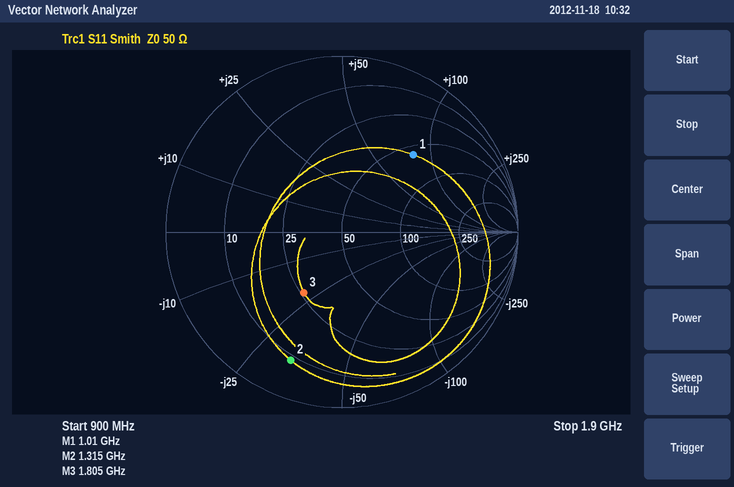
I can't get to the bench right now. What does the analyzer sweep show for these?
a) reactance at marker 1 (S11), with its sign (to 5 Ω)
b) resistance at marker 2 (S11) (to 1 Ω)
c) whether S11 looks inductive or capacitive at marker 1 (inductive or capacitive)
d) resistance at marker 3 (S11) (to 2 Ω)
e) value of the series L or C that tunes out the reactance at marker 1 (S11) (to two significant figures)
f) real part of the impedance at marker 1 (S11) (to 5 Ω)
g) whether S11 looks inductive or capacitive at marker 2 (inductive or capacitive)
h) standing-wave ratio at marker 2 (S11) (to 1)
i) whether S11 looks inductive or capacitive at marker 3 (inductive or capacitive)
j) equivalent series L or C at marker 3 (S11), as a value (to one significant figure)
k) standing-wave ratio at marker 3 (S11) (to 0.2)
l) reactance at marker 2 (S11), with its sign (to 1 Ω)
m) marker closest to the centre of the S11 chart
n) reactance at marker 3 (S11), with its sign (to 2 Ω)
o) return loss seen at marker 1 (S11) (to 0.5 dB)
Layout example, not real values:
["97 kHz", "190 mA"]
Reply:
["+80 Ω", "9 Ω", "inductive", "26 Ω", "2.0 pF", "60 Ω", "capacitive", "8", "capacitive", "4 pF", "2.4", "-33 Ω", "marker 3", "-22 Ω", "4.5 dB"]
